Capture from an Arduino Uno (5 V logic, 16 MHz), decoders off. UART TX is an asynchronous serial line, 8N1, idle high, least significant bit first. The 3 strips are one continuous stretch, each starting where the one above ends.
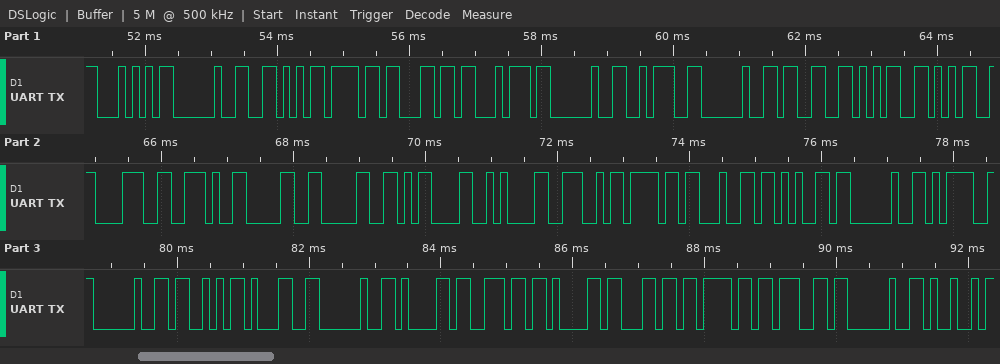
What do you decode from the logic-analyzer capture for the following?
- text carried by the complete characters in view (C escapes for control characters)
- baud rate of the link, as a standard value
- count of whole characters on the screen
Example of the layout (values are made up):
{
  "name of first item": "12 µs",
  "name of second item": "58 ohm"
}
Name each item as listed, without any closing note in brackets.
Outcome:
{
  "text carried by the complete characters in view": "\"T Volt : 3558.00\\r\\nNode = S1 analog I\"",
  "baud rate of the link, as a standard value": "9600 baud",
  "count of whole characters on the screen": "36"
}
